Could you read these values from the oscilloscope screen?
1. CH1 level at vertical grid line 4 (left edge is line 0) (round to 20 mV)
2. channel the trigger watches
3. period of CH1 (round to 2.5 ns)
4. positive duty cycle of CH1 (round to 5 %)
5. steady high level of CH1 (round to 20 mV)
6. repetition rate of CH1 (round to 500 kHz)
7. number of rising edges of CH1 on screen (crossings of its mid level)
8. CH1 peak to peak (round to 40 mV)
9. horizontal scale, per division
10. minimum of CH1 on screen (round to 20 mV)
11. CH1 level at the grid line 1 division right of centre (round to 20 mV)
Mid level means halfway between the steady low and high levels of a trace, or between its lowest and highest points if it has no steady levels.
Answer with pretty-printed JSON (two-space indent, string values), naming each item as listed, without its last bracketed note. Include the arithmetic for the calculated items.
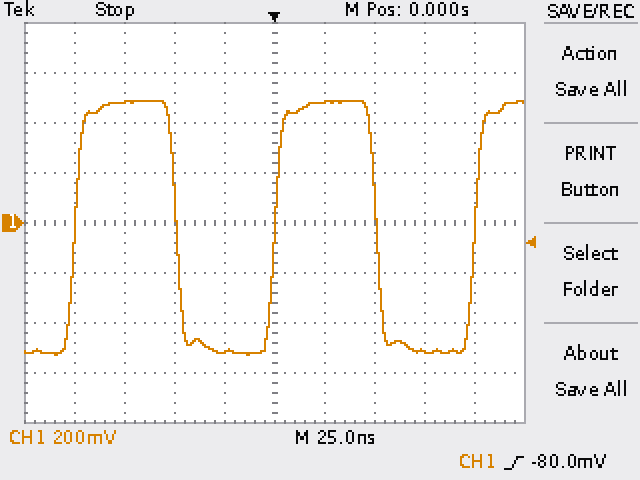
{
  "CH1 level at vertical grid line 4 (left edge is line 0)": "-520 mV",
  "channel the trigger watches": "CH1",
  "period of CH1": "100.0 ns",
  "positive duty cycle of CH1": "50 %",
  "steady high level of CH1": "480 mV",
  "repetition rate of CH1": "1 / 100.0 ns ≈ 10.0 MHz",
  "number of rising edges of CH1 on screen": "3",
  "CH1 peak to peak": "1.00 V",
  "horizontal scale, per division": "25 ns",
  "minimum of CH1 on screen": "-520 mV",
  "CH1 level at the grid line 1 division right of centre": "480 mV"
}
